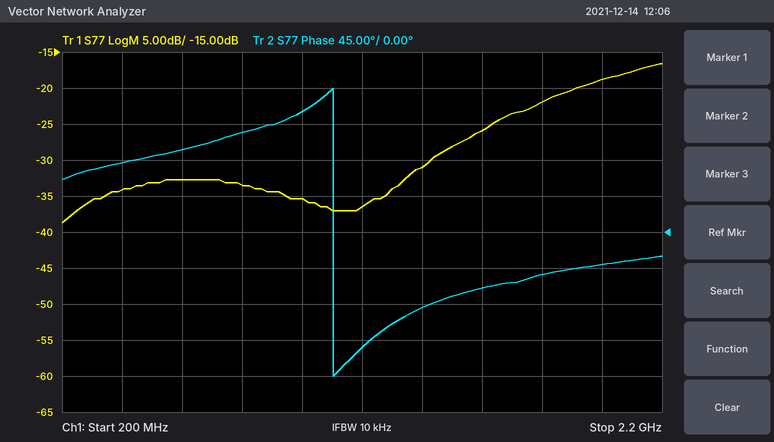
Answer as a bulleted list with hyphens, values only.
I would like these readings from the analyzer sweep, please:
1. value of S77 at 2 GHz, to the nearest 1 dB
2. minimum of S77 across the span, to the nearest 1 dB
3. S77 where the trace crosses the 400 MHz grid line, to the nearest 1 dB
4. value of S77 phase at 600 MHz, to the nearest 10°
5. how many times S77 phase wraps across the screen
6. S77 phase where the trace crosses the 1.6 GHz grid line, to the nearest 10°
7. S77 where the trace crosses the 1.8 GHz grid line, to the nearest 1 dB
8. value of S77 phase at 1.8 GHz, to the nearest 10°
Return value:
- -19 dB
- -39 dB
- -34 dB
- 100°
- 1
- -70°
- -22 dB
- -50°
